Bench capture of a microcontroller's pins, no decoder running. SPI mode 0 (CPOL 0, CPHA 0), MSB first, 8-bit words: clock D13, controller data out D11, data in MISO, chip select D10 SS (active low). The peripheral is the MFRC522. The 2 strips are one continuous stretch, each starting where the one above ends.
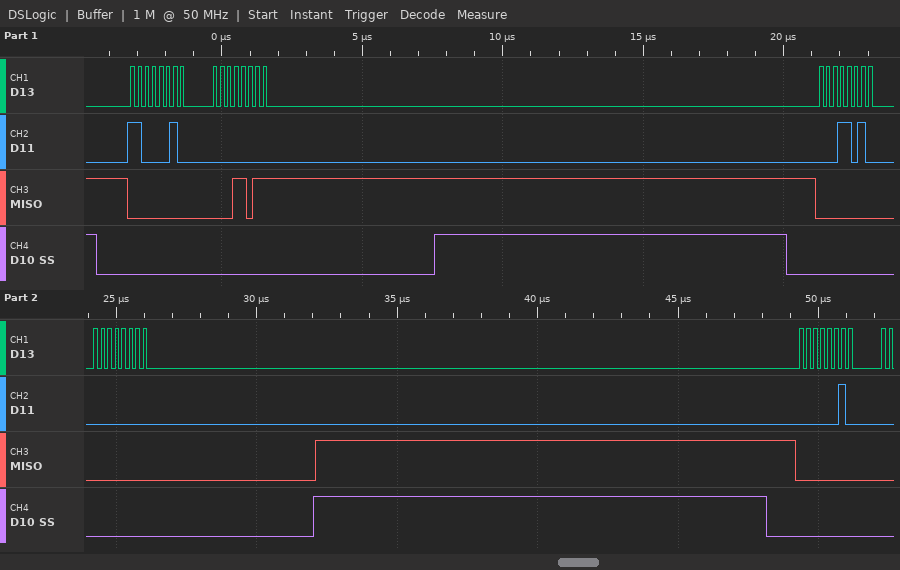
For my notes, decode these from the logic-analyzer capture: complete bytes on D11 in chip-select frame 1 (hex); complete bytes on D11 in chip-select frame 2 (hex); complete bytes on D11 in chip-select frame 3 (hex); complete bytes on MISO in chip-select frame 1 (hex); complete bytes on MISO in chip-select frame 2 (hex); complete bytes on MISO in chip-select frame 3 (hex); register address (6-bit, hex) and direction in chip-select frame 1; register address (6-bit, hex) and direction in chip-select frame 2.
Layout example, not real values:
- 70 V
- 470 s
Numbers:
- C2 00
- 1A 00
- 02
- 00 1B
- 00 00
- 00
- 0x21 read
- 0x0D write
